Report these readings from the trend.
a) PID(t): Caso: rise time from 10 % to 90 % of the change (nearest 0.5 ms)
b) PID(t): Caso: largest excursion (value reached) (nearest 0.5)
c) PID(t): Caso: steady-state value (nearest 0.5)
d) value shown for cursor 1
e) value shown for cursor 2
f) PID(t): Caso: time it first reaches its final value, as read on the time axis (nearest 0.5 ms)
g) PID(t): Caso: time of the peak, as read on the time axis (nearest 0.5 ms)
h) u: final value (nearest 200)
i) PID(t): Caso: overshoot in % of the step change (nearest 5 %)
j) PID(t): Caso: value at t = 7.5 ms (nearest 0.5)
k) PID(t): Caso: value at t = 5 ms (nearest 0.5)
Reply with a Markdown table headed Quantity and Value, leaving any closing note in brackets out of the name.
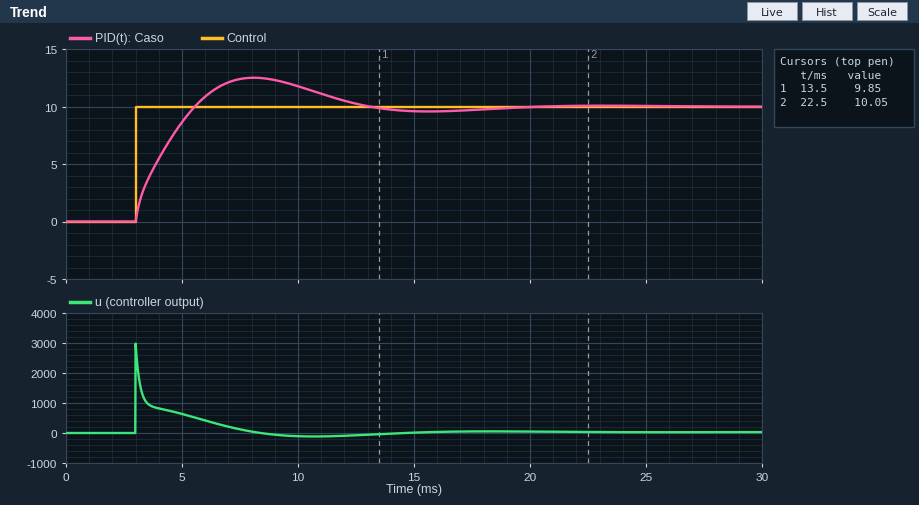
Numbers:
| Quantity | Value |
|---|---|
| PID(t): Caso: rise time from 10 % to 90 % of the change | 2.0 ms |
| PID(t): Caso: largest excursion (value reached) | 12.5 |
| PID(t): Caso: steady-state value | 10.0 |
| value shown for cursor 1 | 9.85 |
| value shown for cursor 2 | 10.05 |
| PID(t): Caso: time it first reaches its final value, as read on the time axis | 5.5 ms |
| PID(t): Caso: time of the peak, as read on the time axis | 8.0 ms |
| u: final value | 0 |
| PID(t): Caso: overshoot in % of the step change | 25 % |
| PID(t): Caso: value at t = 7.5 ms | 12.5 |
| PID(t): Caso: value at t = 5 ms | 8.5 |
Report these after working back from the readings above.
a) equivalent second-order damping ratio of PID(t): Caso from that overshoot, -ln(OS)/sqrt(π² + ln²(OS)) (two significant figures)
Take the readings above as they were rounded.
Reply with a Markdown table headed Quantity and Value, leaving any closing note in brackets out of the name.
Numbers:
| Quantity | Value |
|---|---|
| equivalent second-order damping ratio of PID(t): Caso from that overshoot, -ln(OS)/sqrt(π² + ln²(OS)) | 0.40 |
